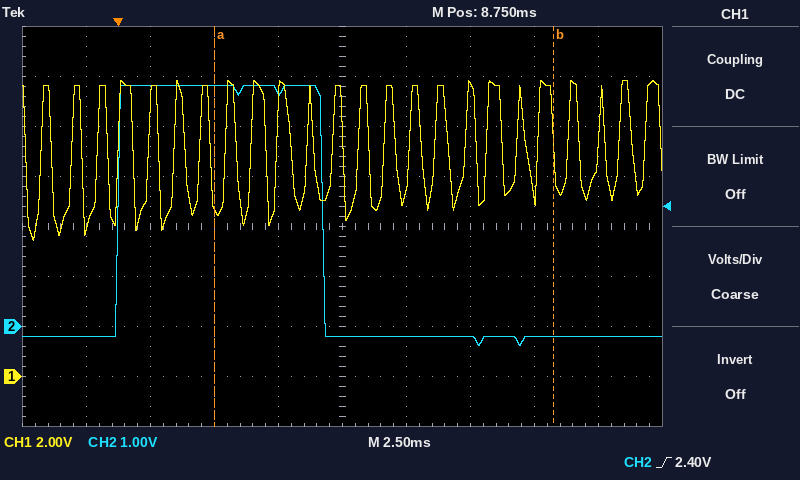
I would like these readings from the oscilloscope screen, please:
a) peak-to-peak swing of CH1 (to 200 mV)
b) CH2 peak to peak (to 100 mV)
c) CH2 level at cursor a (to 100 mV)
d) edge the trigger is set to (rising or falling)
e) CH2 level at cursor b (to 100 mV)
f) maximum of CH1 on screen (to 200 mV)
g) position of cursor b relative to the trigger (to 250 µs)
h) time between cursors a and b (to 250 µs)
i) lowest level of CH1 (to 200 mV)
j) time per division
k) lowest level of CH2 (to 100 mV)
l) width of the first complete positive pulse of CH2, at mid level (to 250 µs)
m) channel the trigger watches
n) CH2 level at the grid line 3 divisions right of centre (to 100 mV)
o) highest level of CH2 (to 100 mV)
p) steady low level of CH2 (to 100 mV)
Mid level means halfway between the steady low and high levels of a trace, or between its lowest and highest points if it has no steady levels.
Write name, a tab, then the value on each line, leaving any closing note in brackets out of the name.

peak-to-peak swing of CH1	6.4 V
CH2 peak to peak	5.2 V
CH2 level at cursor a	4.8 V
edge the trigger is set to	rising
CH2 level at cursor b	-200 mV
maximum of CH1 on screen	11.8 V
position of cursor b relative to the trigger	+17.00 ms
time between cursors a and b	13.25 ms
lowest level of CH1	5.4 V
time per division	2.5 ms
lowest level of CH2	-400 mV
width of the first complete positive pulse of CH2, at mid level	8.00 ms
channel the trigger watches	CH2
CH2 level at the grid line 3 divisions right of centre	-200 mV
highest level of CH2	4.8 V
steady low level of CH2	-200 mV
